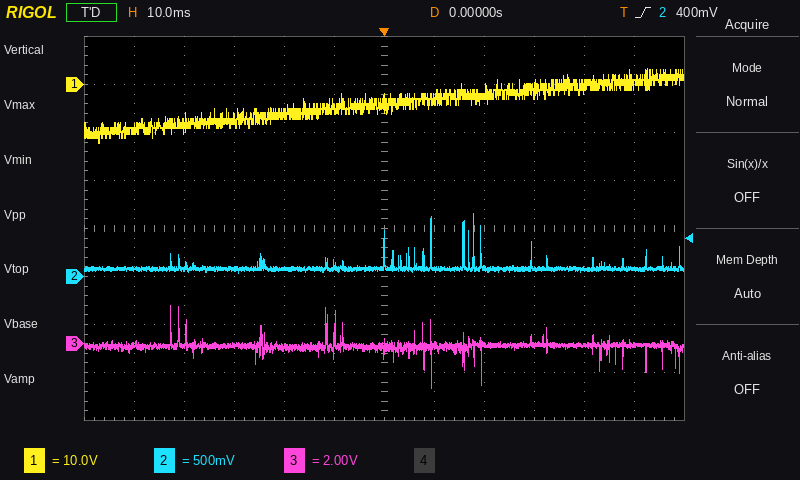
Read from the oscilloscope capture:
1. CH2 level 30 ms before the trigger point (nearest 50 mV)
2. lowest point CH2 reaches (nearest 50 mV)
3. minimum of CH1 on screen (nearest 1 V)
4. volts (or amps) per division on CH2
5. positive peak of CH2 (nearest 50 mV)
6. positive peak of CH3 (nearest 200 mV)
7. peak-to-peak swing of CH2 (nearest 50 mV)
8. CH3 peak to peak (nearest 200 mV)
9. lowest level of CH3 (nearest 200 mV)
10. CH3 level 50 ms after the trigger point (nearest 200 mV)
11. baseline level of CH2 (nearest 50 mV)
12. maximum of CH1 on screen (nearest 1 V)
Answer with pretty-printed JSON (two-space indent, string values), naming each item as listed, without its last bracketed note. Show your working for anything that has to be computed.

{
  "CH2 level 30 ms before the trigger point": "100 mV",
  "lowest point CH2 reaches": "50 mV",
  "minimum of CH1 on screen": "-12 V",
  "volts (or amps) per division on CH2": "500 mV",
  "positive peak of CH2": "650 mV",
  "positive peak of CH3": "1.6 V",
  "peak-to-peak swing of CH2": "650 mV − (50 mV) = 600 mV",
  "CH3 peak to peak": "1.6 V − (-1.8 V) = 3.4 V",
  "lowest level of CH3": "-1.8 V",
  "CH3 level 50 ms after the trigger point": "0.0 V",
  "baseline level of CH2": "100 mV",
  "maximum of CH1 on screen": "3 V"
}
